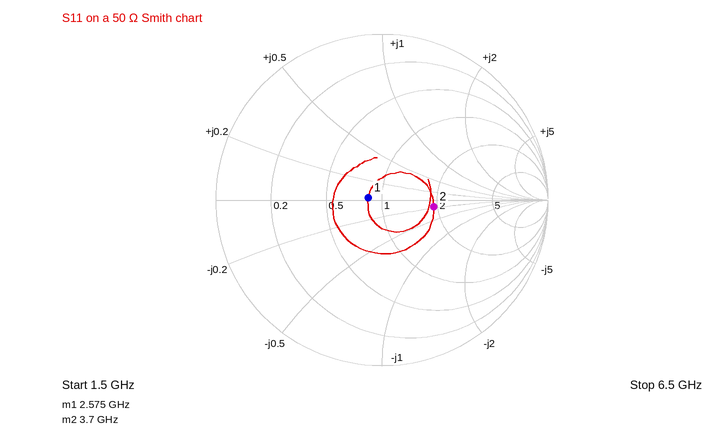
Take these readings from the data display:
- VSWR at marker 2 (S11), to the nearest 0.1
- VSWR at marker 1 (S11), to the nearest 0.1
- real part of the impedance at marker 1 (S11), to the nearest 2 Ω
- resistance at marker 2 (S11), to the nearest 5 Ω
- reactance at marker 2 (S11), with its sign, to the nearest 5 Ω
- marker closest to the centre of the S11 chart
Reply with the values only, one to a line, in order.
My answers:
1.9
1.2
42 Ω
95 Ω
-10 Ω
marker 1
